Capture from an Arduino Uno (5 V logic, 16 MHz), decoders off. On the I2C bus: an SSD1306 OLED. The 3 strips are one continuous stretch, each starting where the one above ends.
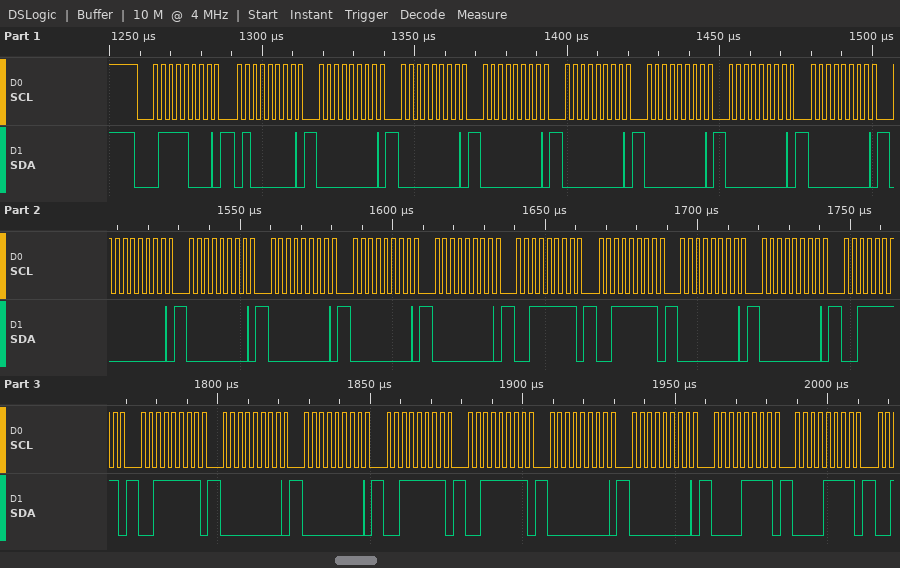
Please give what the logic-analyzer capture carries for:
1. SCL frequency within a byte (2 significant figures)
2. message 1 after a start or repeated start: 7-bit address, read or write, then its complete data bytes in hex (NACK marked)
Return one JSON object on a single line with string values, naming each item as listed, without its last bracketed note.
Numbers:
{"SCL frequency within a byte": "400 kHz", "message 1 after a start or repeated start: 7-bit address, read or write, then its complete data bytes in hex": "0x3C write: 40 00 00 00 00 00 00 00 00 00 00 00 00 3F 3F 00 00 3F 3F 00 00 3F 3F 00 00 0F 0F"}
